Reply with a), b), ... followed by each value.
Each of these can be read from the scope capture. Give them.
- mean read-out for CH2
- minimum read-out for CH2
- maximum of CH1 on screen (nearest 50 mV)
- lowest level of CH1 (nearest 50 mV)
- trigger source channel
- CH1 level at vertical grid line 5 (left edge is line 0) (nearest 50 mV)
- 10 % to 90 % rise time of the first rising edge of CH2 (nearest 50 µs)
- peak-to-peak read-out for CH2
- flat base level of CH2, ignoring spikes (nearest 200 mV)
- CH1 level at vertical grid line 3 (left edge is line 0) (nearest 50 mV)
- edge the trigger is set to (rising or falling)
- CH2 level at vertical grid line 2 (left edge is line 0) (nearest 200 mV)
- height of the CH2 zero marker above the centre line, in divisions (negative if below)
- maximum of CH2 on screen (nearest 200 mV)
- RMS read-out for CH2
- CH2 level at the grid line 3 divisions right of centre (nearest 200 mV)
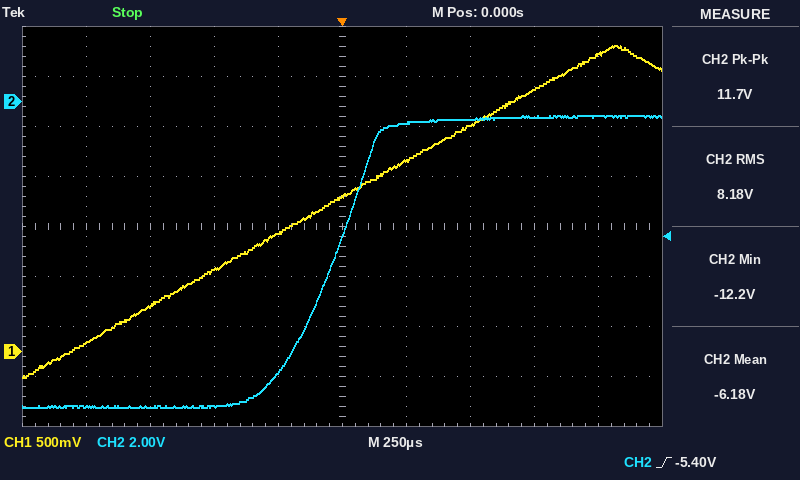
a) -6.18 V
b) -12.2 V
c) 3.05 V
d) -250 mV
e) CH2
f) 1.55 V
g) 400 µs
h) 11.7 V
i) -12.2 V
j) 800 mV
k) rising
l) -12.2 V
m) +2.5 div
n) -600 mV
o) 8.18 V
p) -600 mV
